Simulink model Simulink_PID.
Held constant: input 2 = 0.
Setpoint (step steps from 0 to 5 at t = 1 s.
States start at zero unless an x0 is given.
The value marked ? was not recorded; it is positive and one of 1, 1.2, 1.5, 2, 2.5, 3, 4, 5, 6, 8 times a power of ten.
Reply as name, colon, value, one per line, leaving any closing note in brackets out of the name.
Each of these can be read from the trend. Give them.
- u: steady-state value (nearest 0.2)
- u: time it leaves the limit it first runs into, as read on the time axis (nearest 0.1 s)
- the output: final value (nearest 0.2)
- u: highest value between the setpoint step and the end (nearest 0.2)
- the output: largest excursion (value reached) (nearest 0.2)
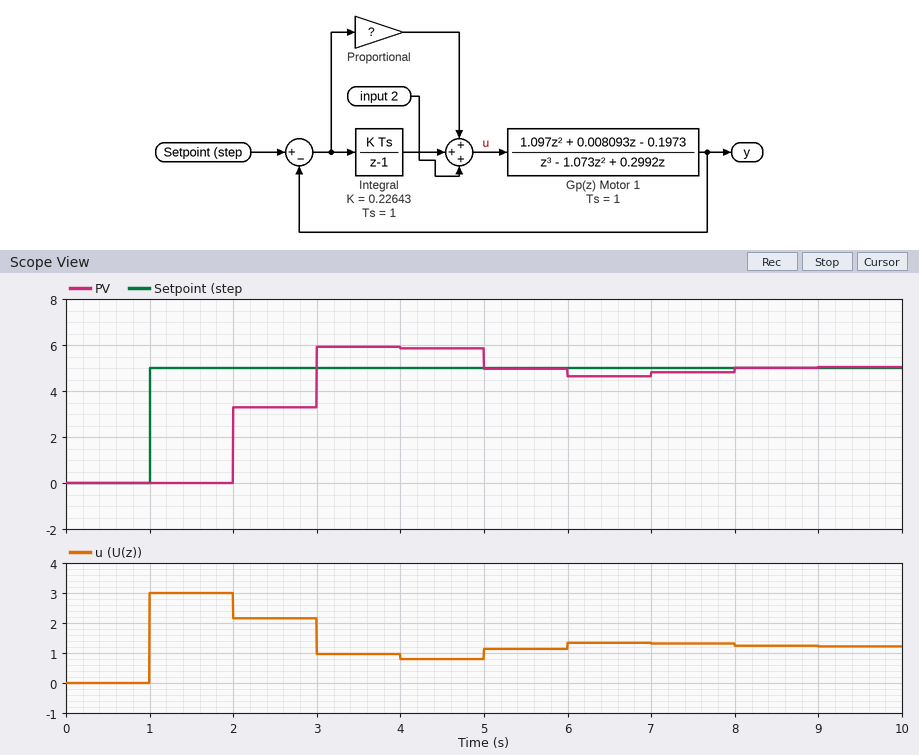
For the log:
u: steady-state value: 1.2
u: time it leaves the limit it first runs into, as read on the time axis: 2.0 s
the output: final value: 5.0
u: highest value between the setpoint step and the end: 3.0
the output: largest excursion (value reached): 6.0
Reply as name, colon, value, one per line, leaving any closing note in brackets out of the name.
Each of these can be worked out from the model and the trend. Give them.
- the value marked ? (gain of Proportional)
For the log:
the value marked ?: 0.6
